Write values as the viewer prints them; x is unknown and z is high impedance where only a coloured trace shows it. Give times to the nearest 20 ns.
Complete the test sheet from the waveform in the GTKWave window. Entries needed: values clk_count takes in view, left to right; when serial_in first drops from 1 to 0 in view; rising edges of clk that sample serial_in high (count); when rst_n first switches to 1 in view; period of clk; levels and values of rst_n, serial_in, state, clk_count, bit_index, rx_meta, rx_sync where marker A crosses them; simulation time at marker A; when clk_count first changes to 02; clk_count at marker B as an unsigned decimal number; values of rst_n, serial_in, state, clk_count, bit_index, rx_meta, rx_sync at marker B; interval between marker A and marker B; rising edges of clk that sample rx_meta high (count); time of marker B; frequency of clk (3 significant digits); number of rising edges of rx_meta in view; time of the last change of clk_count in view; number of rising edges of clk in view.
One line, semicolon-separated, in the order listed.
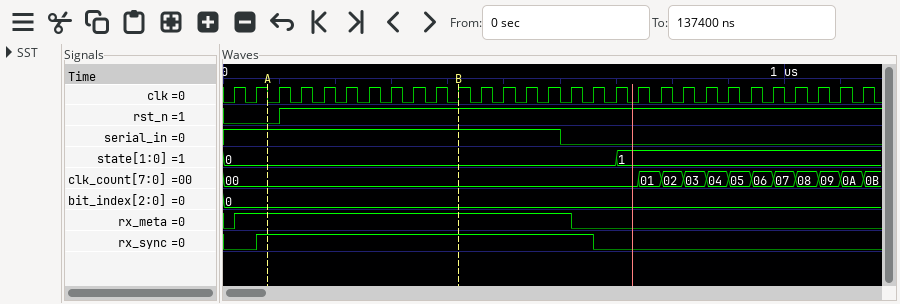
00, 01, 02, 03, 04, 05, 06, 07, 08, 09, 0A, 0B; 600 ns; 15; 100 ns; 40 ns; rst_n=0, serial_in=1, state=0, clk_count=00, bit_index=0, rx_meta=1, rx_sync=1; 80 ns; 780 ns; 0; rst_n=1, serial_in=1, state=0, clk_count=00, bit_index=0, rx_meta=1, rx_sync=1; 340 ns; 15; 420 ns; 25.0 MHz; 1; 1140 ns; 29
